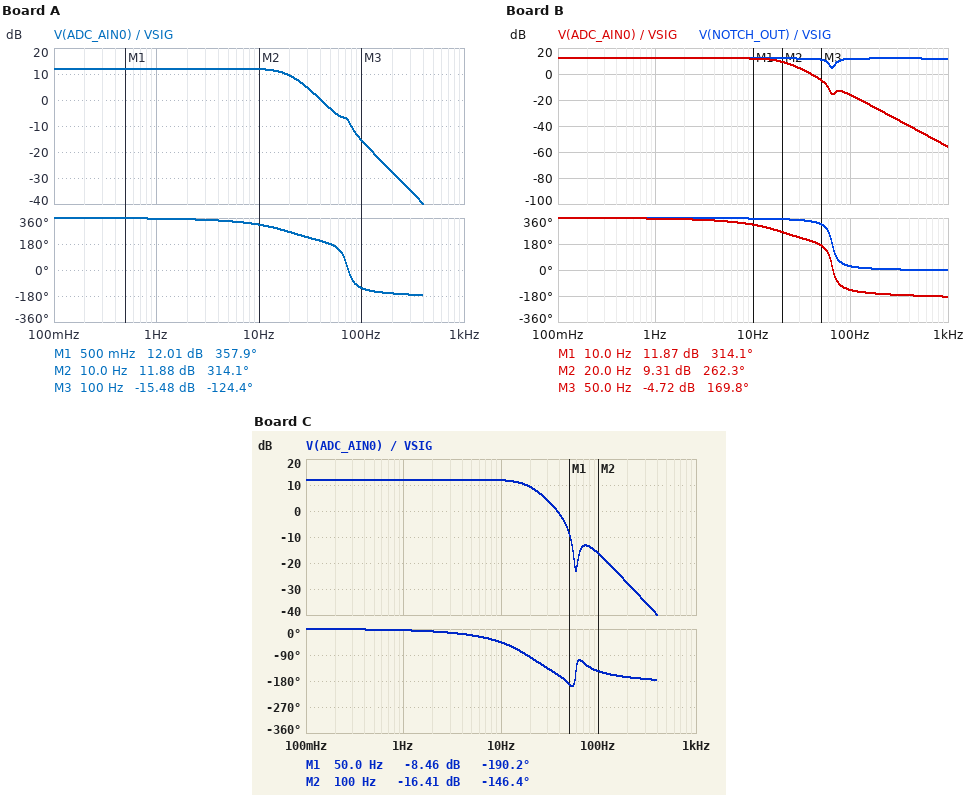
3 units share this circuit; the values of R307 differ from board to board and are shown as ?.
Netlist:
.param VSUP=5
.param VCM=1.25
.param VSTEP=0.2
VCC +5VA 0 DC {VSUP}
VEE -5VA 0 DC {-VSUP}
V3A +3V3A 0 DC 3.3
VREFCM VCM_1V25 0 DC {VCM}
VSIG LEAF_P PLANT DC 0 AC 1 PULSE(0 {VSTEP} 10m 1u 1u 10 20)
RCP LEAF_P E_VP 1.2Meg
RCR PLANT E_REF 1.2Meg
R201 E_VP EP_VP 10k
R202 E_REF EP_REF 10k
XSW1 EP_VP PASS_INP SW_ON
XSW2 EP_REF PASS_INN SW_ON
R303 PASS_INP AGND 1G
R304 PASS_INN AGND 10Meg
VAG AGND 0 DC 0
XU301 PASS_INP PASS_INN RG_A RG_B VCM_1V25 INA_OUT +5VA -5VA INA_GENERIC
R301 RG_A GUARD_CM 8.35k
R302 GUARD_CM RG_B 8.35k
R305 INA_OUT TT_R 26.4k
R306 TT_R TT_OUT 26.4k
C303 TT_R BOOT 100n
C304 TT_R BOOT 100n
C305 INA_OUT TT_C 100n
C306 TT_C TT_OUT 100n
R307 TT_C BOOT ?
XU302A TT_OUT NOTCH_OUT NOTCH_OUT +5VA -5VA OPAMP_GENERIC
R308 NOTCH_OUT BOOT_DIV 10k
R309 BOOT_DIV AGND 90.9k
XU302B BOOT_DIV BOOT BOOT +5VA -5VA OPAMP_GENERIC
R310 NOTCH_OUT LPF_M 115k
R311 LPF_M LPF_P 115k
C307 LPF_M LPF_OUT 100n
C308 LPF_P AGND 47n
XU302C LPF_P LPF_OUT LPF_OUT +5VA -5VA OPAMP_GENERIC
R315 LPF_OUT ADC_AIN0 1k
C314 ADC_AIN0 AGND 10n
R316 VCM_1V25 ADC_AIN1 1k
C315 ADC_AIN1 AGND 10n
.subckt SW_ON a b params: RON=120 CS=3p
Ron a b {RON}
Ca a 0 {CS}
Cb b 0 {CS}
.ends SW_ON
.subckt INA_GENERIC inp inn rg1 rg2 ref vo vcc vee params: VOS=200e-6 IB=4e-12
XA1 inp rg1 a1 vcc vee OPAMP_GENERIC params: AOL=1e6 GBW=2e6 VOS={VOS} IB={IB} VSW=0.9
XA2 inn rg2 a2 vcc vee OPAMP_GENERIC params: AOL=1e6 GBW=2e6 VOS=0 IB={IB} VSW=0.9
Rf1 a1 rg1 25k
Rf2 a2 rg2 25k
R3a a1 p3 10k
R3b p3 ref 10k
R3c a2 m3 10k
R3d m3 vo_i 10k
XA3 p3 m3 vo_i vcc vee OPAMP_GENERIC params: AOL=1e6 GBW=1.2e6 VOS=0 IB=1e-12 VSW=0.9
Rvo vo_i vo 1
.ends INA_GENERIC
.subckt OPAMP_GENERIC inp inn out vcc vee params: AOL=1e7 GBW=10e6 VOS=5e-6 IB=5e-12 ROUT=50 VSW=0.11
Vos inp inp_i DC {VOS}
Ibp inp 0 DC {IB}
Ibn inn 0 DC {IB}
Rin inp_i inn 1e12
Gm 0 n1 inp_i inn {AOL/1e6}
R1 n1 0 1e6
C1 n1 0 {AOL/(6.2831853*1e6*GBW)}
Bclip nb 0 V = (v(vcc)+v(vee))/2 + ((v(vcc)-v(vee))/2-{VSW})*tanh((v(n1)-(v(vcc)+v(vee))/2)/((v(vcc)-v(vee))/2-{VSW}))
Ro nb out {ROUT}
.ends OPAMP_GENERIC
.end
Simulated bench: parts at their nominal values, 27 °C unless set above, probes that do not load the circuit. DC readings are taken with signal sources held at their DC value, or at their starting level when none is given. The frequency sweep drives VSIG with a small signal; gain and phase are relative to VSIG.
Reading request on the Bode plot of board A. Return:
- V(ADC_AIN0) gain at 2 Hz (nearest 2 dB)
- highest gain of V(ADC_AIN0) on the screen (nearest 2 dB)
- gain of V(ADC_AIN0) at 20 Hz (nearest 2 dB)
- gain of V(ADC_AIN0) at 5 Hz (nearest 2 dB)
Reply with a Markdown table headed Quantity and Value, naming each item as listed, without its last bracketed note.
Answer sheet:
| Quantity | Value |
|---|---|
| V(ADC_AIN0) gain at 2 Hz | 12 dB |
| highest gain of V(ADC_AIN0) on the screen | 12 dB |
| gain of V(ADC_AIN0) at 20 Hz | 10 dB |
| gain of V(ADC_AIN0) at 5 Hz | 12 dB |
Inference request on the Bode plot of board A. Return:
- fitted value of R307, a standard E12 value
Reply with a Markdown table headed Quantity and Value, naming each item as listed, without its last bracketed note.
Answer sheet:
| Quantity | Value |
|---|---|
| fitted value of R307, a standard E12 value | 6.8 kΩ |
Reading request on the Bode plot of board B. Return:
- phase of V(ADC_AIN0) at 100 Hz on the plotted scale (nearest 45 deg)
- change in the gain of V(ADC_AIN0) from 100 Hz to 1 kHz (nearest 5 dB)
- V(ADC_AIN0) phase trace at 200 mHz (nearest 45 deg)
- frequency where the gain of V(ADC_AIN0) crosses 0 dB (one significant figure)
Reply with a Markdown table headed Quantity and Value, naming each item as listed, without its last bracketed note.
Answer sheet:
| Quantity | Value |
|---|---|
| phase of V(ADC_AIN0) at 100 Hz on the plotted scale | -135 deg |
| change in the gain of V(ADC_AIN0) from 100 Hz to 1 kHz | -40 dB |
| V(ADC_AIN0) phase trace at 200 mHz | 360 deg |
| frequency where the gain of V(ADC_AIN0) crosses 0 dB | 40 Hz |
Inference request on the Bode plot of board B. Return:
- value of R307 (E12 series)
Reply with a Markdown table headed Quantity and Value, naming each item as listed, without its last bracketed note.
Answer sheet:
| Quantity | Value |
|---|---|
| value of R307 | 10 kΩ |
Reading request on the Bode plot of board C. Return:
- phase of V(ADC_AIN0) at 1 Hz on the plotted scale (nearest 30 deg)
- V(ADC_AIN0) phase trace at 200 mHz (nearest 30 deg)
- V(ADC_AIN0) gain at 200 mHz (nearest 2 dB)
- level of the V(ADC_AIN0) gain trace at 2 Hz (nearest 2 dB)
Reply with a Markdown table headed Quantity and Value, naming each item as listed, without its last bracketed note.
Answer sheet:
| Quantity | Value |
|---|---|
| phase of V(ADC_AIN0) at 1 Hz on the plotted scale | 0 deg |
| V(ADC_AIN0) phase trace at 200 mHz | 0 deg |
| V(ADC_AIN0) gain at 200 mHz | 12 dB |
| level of the V(ADC_AIN0) gain trace at 2 Hz | 12 dB |
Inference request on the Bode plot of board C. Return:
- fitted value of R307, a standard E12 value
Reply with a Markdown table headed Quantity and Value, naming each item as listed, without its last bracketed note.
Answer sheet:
| Quantity | Value |
|---|---|
| fitted value of R307, a standard E12 value | 15 kΩ |
